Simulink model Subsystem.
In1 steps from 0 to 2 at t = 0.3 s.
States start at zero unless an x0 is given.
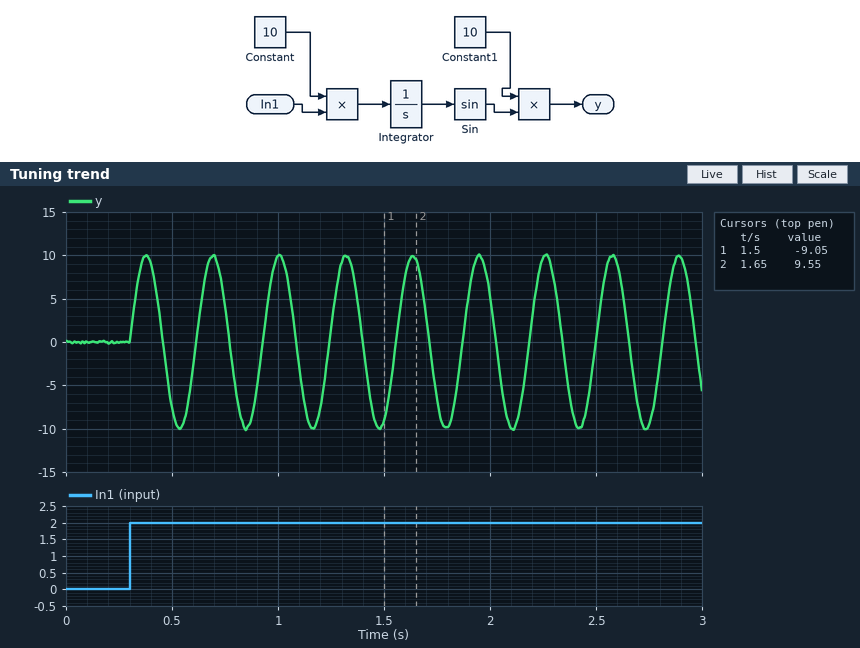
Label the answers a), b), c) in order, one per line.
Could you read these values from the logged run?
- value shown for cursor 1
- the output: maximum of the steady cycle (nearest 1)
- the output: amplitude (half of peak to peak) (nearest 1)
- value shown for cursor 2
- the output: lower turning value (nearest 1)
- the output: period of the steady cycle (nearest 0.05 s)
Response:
a) -9.05
b) 10
c) 10
d) 9.55
e) -10
f) 0.30 s
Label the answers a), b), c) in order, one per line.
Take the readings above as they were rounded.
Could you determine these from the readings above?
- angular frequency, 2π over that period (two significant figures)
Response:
a) 21 rad/s
